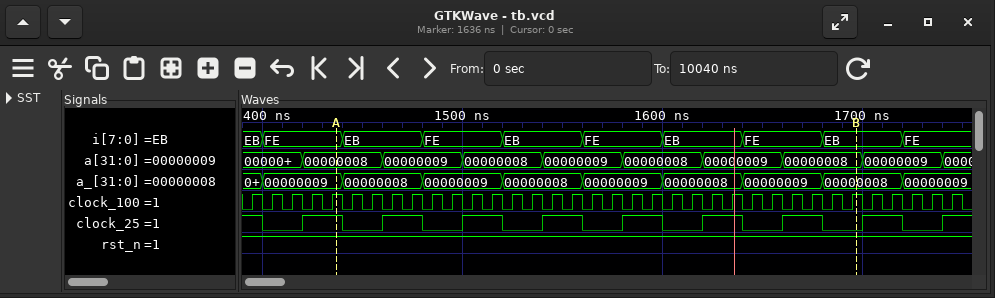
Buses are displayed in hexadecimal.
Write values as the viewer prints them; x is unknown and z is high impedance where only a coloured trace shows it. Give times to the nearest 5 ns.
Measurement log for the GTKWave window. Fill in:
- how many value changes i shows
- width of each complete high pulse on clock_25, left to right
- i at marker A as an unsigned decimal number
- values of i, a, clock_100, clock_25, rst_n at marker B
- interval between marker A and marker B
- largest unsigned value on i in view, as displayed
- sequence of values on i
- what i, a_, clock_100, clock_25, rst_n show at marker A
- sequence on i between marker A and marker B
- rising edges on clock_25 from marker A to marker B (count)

9
20 ns, 20 ns, 20 ns, 20 ns, 20 ns, 20 ns, 20 ns, 20 ns
254
i=EB, a=00000008, clock_100=1, clock_25=0, rst_n=1
260 ns
FE
EB, FE, EB, FE, EB, FE, EB, FE, EB, FE
i=FE, a_=00000009, clock_100=1, clock_25=1, rst_n=1
FE, EB, FE, EB, FE, EB, FE, EB
6
